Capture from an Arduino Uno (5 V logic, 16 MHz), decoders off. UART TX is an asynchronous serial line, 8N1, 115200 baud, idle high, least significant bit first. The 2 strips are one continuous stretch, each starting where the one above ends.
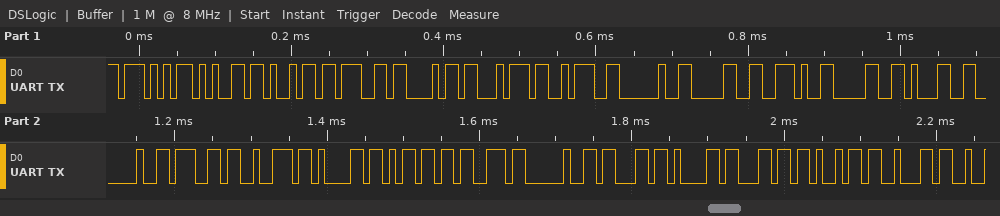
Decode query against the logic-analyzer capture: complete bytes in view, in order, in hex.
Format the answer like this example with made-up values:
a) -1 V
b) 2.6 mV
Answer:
a) 0x57 0x65 0x69 0x67 0x68 0x74 0x3A 0x20 0x30 0x2E 0x30 0x31 0x20 0x67 0x72 0x61 0x6D 0x73 0x20 0x63 0x61 0x6C 0x69 0x62
